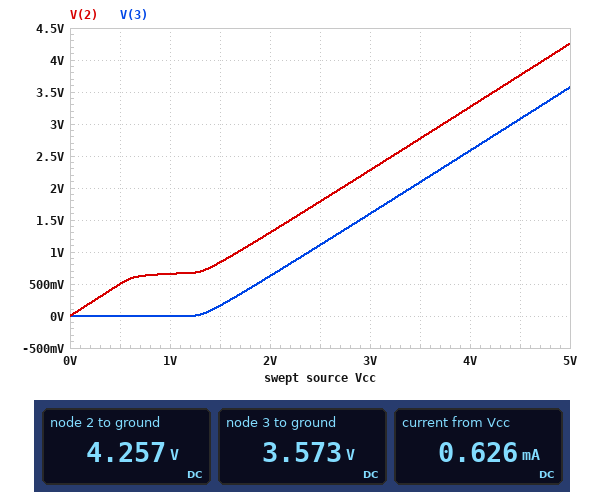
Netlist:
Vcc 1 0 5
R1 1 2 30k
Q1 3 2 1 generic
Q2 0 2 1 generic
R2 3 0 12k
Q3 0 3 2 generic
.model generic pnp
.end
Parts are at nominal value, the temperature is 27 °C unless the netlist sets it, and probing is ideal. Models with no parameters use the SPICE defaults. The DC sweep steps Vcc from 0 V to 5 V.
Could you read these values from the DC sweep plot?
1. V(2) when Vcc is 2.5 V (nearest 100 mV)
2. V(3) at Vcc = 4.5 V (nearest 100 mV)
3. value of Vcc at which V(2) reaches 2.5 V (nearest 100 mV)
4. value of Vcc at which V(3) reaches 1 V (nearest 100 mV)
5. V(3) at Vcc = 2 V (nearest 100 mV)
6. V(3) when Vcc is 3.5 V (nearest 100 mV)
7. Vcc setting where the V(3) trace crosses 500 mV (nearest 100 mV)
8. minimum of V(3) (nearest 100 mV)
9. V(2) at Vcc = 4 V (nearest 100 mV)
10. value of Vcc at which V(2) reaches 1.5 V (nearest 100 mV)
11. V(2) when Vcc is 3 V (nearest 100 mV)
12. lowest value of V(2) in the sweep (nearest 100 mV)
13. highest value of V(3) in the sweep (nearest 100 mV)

1.8 V
3.1 V
3.2 V
2.4 V
600 mV
2.1 V
1.9 V
0 V
3.3 V
2.2 V
2.3 V
0 V
3.6 V
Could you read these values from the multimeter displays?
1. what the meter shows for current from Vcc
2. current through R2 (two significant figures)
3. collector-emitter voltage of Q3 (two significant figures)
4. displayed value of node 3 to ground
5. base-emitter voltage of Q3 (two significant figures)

0.626 mA
300 µA
-4.3 V
3.573 V
-680 mV
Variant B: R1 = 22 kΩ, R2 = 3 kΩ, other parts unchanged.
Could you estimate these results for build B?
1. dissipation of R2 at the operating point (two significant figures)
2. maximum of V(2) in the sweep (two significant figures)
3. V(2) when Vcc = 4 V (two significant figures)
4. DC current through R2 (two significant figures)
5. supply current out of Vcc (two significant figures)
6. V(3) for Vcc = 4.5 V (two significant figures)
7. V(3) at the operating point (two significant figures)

4.1 mW
4.2 V
3.2 V
1.2 mA
2.4 mA
3.0 V
3.5 V
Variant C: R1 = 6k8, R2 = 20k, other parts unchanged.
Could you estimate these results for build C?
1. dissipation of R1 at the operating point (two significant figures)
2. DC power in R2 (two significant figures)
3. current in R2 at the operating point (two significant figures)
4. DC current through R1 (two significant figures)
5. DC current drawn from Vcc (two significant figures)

78 µW
630 µW
180 µA
110 µA
460 µA
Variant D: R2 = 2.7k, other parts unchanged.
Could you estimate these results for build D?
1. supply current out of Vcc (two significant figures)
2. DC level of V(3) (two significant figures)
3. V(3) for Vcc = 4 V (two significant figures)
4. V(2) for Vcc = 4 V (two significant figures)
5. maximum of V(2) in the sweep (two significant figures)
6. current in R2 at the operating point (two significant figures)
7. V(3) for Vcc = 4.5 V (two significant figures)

2.7 mA
3.5 V
2.5 V
3.2 V
4.2 V
1.3 mA
3.0 V
